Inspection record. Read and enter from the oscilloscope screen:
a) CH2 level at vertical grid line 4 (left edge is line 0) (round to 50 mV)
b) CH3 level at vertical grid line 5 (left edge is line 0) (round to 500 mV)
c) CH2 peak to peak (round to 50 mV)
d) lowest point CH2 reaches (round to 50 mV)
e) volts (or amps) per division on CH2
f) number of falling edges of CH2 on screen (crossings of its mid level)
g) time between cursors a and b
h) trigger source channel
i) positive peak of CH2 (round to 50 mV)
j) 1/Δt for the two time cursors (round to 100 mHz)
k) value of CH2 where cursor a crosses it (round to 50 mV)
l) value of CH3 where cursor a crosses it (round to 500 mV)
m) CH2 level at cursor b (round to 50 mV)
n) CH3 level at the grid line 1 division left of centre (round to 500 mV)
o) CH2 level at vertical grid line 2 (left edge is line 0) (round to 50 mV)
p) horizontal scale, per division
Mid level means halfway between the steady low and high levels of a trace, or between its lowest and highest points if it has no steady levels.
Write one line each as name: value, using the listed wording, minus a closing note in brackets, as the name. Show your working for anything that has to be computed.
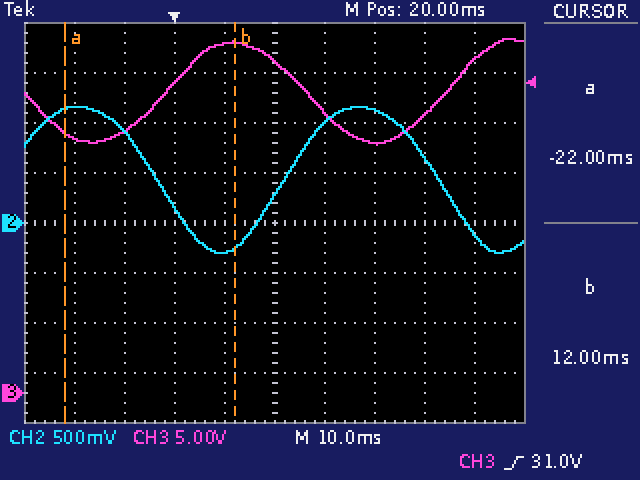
CH2 level at vertical grid line 4 (left edge is line 0): -300 mV
CH3 level at vertical grid line 5 (left edge is line 0): 33.0 V
CH2 peak to peak: 1.15 V − (-300 mV) = 1.45 V
lowest point CH2 reaches: -300 mV
volts (or amps) per division on CH2: 500 mV
number of falling edges of CH2 on screen: 2
time between cursors a and b: 12 ms − (-22 ms) = 34 ms
trigger source channel: CH3
positive peak of CH2: 1.15 V
1/Δt for the two time cursors: 1 / 34 ms ≈ 29.4 Hz
value of CH2 where cursor a crosses it: 1.15 V
value of CH3 where cursor a crosses it: 26.0 V
CH2 level at cursor b: -250 mV
CH3 level at the grid line 1 division left of centre: 35.0 V
CH2 level at vertical grid line 2 (left edge is line 0): 900 mV
horizontal scale, per division: 10 ms
